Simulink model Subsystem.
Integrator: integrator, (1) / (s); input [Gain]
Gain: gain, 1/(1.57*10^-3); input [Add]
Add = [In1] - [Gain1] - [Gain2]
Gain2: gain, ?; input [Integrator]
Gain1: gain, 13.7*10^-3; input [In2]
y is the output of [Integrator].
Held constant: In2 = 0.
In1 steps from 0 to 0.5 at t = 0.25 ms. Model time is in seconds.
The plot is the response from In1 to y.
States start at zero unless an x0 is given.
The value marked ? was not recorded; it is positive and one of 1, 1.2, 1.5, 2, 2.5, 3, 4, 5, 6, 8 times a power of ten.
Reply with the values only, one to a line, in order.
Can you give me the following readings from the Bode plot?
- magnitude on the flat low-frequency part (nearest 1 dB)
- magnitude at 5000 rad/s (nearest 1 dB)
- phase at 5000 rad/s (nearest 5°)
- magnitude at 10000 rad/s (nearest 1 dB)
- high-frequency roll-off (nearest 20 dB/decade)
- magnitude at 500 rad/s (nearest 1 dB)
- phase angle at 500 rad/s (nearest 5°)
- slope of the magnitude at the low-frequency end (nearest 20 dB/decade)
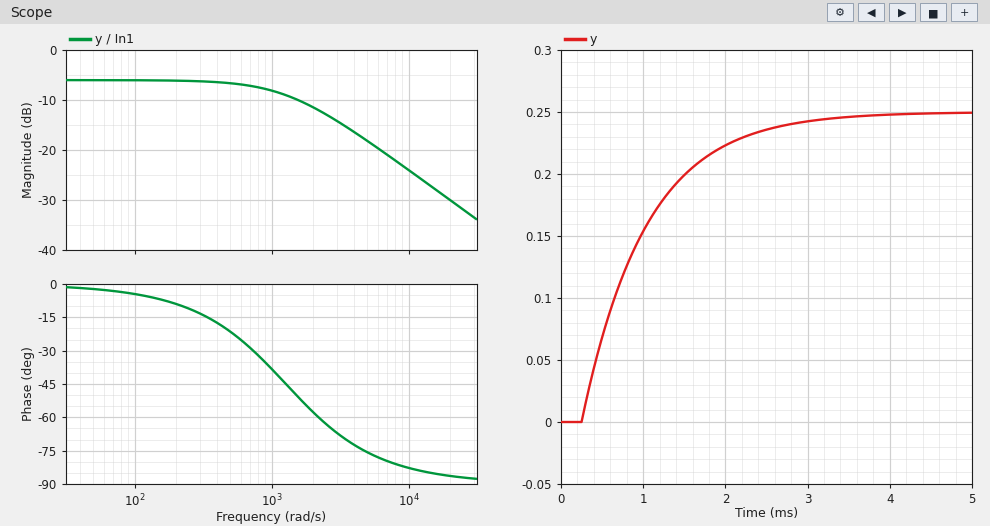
-6 dB
-18 dB
-75°
-24 dB
-20 dB/decade
-7 dB
-20°
0 dB/decade
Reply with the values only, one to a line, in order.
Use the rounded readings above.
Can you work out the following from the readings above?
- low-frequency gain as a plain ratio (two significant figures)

0.50
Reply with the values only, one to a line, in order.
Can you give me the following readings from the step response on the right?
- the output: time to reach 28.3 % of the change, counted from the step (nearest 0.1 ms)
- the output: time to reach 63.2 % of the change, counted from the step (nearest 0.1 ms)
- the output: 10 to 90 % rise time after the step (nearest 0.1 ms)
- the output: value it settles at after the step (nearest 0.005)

0.3 ms
0.8 ms
1.7 ms
0.250
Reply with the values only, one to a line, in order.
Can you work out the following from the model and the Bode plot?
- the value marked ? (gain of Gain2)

2
